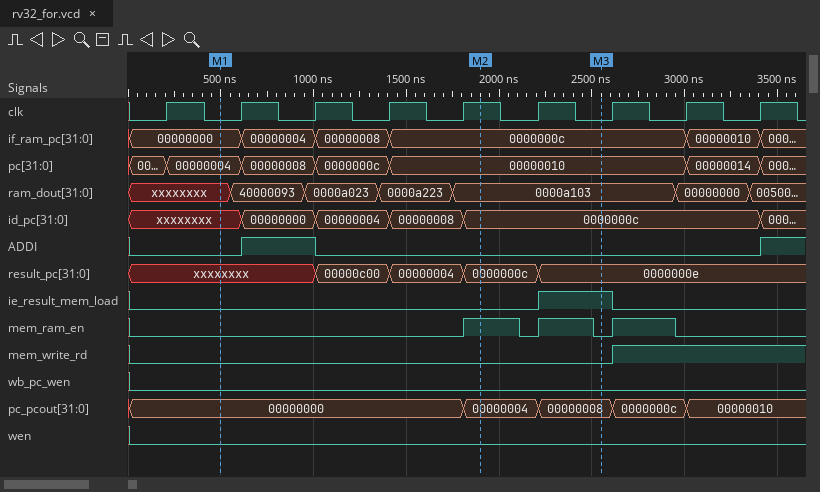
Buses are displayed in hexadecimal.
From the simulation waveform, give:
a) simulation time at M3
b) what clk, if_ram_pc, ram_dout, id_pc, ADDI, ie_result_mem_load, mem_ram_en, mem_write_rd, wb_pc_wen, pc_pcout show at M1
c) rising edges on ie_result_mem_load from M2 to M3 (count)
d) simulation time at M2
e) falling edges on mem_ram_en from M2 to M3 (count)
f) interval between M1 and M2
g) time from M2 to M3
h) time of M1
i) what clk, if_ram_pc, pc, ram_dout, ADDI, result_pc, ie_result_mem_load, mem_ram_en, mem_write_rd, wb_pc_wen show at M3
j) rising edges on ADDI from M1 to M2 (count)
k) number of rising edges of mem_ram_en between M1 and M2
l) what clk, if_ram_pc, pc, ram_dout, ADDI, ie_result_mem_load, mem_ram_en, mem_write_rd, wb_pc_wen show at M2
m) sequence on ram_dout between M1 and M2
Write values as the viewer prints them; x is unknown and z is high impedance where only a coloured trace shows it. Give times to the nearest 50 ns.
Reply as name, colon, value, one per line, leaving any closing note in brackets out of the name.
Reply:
simulation time at M3: 2550 ns
what clk, if_ram_pc, ram_dout, id_pc, ADDI, ie_result_mem_load, mem_ram_en, mem_write_rd, wb_pc_wen, pc_pcout show at M1: clk=0, if_ram_pc=00000000, ram_dout=xxxxxxxx, id_pc=xxxxxxxx, ADDI=0, ie_result_mem_load=0, mem_ram_en=0, mem_write_rd=0, wb_pc_wen=0, pc_pcout=00000000
rising edges on ie_result_mem_load from M2 to M3: 1
simulation time at M2: 1900 ns
falling edges on mem_ram_en from M2 to M3: 2
interval between M1 and M2: 1400 ns
time from M2 to M3: 650 ns
time of M1: 500 ns
what clk, if_ram_pc, pc, ram_dout, ADDI, result_pc, ie_result_mem_load, mem_ram_en, mem_write_rd, wb_pc_wen show at M3: clk=0, if_ram_pc=0000000c, pc=00000010, ram_dout=0000a103, ADDI=0, result_pc=0000000e, ie_result_mem_load=1, mem_ram_en=0, mem_write_rd=0, wb_pc_wen=0
rising edges on ADDI from M1 to M2: 1
number of rising edges of mem_ram_en between M1 and M2: 1
what clk, if_ram_pc, pc, ram_dout, ADDI, ie_result_mem_load, mem_ram_en, mem_write_rd, wb_pc_wen show at M2: clk=1, if_ram_pc=0000000c, pc=00000010, ram_dout=0000a103, ADDI=0, ie_result_mem_load=0, mem_ram_en=1, mem_write_rd=0, wb_pc_wen=0
sequence on ram_dout between M1 and M2: xxxxxxxx, 40000093, 0000a023, 0000a223, 0000a103
